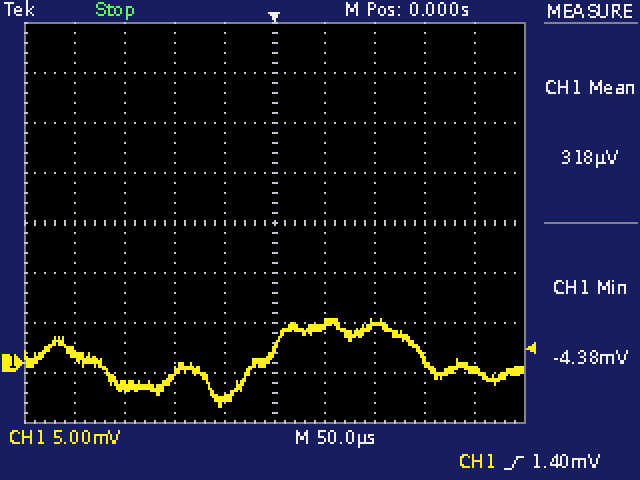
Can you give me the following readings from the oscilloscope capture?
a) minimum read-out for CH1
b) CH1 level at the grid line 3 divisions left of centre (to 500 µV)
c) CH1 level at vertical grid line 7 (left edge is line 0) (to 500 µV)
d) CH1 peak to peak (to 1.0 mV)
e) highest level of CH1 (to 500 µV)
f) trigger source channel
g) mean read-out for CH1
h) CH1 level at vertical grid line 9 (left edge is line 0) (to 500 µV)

-4.38 mV
-2.5 mV
4.0 mV
9.0 mV
4.5 mV
CH1
318 µV
-500 µV
